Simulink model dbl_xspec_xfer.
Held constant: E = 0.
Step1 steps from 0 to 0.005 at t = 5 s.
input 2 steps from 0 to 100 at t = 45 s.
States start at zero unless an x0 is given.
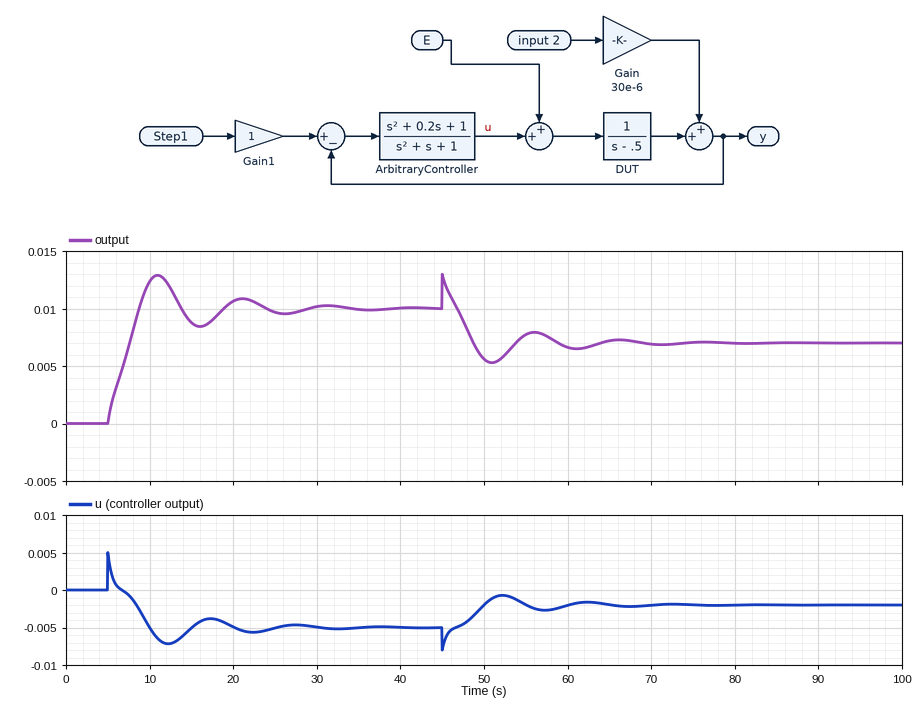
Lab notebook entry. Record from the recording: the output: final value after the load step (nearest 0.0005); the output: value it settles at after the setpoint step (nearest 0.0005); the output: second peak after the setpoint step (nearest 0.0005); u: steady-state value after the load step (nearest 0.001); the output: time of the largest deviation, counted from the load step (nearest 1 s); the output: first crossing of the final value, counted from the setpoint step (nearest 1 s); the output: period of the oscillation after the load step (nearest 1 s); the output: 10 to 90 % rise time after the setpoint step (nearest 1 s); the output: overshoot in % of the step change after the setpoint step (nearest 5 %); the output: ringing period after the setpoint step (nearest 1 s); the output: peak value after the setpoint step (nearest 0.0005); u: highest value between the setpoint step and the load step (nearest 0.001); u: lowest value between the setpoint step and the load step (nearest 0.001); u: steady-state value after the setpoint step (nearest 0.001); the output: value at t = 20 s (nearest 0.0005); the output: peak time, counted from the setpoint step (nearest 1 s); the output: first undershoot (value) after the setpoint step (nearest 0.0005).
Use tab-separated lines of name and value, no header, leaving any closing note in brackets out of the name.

the output: final value after the load step	0.0070
the output: value it settles at after the setpoint step	0.0100
the output: second peak after the setpoint step	0.0110
u: steady-state value after the load step	-0.002
the output: time of the largest deviation, counted from the load step	6 s
the output: first crossing of the final value, counted from the setpoint step	4 s
the output: period of the oscillation after the load step	10 s
the output: 10 to 90 % rise time after the setpoint step	3 s
the output: overshoot in % of the step change after the setpoint step	30 %
the output: ringing period after the setpoint step	10 s
the output: peak value after the setpoint step	0.0130
u: highest value between the setpoint step and the load step	0.005
u: lowest value between the setpoint step and the load step	-0.007
u: steady-state value after the setpoint step	-0.005
the output: value at t = 20 s	0.0105
the output: peak time, counted from the setpoint step	6 s
the output: first undershoot (value) after the setpoint step	0.0085
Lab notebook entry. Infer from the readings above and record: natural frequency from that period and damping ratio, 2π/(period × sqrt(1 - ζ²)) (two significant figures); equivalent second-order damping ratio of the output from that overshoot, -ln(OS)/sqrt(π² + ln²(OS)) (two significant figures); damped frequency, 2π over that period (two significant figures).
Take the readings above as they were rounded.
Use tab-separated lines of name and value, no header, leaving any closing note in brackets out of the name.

natural frequency from that period and damping ratio, 2π/(period × sqrt(1 - ζ²))	0.67 rad/s
equivalent second-order damping ratio of the output from that overshoot, -ln(OS)/sqrt(π² + ln²(OS))	0.36
damped frequency, 2π over that period	0.63 rad/s
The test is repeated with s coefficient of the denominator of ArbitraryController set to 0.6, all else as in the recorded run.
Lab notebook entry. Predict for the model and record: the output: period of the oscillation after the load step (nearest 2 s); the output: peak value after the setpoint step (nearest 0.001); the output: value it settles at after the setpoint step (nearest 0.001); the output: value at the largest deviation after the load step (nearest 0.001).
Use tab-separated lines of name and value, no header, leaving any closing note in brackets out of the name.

the output: period of the oscillation after the load step	8 s
the output: peak value after the setpoint step	0.011
the output: value it settles at after the setpoint step	0.010
the output: value at the largest deviation after the load step	0.006
